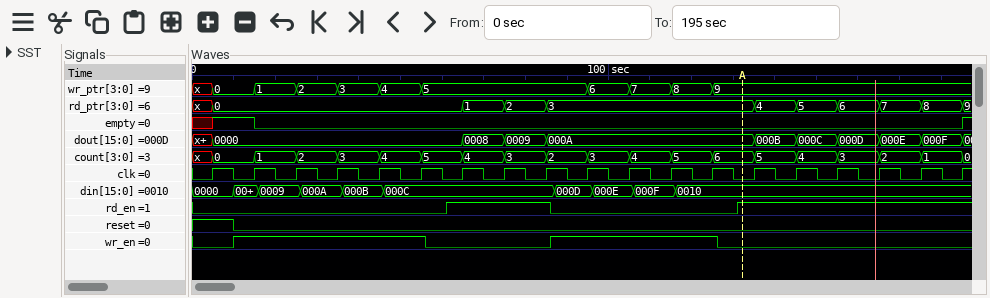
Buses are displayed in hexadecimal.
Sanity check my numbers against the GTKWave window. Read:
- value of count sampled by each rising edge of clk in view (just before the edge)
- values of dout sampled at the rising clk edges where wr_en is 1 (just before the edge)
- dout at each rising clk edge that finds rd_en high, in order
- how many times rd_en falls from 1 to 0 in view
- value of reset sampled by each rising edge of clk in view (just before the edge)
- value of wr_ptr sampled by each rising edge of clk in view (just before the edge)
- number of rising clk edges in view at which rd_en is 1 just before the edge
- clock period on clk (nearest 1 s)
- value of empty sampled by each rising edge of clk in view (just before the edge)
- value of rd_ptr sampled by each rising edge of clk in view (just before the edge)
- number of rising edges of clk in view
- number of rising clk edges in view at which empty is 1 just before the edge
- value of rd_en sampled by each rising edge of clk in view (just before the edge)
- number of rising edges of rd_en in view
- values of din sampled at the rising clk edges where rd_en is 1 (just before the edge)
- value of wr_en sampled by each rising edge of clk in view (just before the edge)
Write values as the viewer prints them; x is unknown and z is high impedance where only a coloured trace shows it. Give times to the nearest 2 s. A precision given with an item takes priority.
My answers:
x, 0, 1, 2, 3, 4, 5, 4, 3, 2, 3, 4, 5, 6, 5, 4, 3, 2, 1
0000, 0000, 0000, 0000, 0000, 000A, 000A, 000A, 000A
0000, 0008, 0009, 000A, 000B, 000C, 000D, 000E, 000F
1
1 0 0 0 0 0 0 0 0 0 0 0 0 0 0 0 0 0 0
x, 0, 1, 2, 3, 4, 5, 5, 5, 5, 6, 7, 8, 9, 9, 9, 9, 9, 9
9
10 s
x 1 0 0 0 0 0 0 0 0 0 0 0 0 0 0 0 0 0
x, 0, 0, 0, 0, 0, 0, 1, 2, 3, 3, 3, 3, 3, 4, 5, 6, 7, 8
19
1
0 0 0 0 0 0 1 1 1 0 0 0 0 1 1 1 1 1 1
2
000C, 000C, 000C, 0010, 0010, 0010, 0010, 0010, 0010
0 1 1 1 1 1 0 0 0 1 1 1 1 0 0 0 0 0 0
